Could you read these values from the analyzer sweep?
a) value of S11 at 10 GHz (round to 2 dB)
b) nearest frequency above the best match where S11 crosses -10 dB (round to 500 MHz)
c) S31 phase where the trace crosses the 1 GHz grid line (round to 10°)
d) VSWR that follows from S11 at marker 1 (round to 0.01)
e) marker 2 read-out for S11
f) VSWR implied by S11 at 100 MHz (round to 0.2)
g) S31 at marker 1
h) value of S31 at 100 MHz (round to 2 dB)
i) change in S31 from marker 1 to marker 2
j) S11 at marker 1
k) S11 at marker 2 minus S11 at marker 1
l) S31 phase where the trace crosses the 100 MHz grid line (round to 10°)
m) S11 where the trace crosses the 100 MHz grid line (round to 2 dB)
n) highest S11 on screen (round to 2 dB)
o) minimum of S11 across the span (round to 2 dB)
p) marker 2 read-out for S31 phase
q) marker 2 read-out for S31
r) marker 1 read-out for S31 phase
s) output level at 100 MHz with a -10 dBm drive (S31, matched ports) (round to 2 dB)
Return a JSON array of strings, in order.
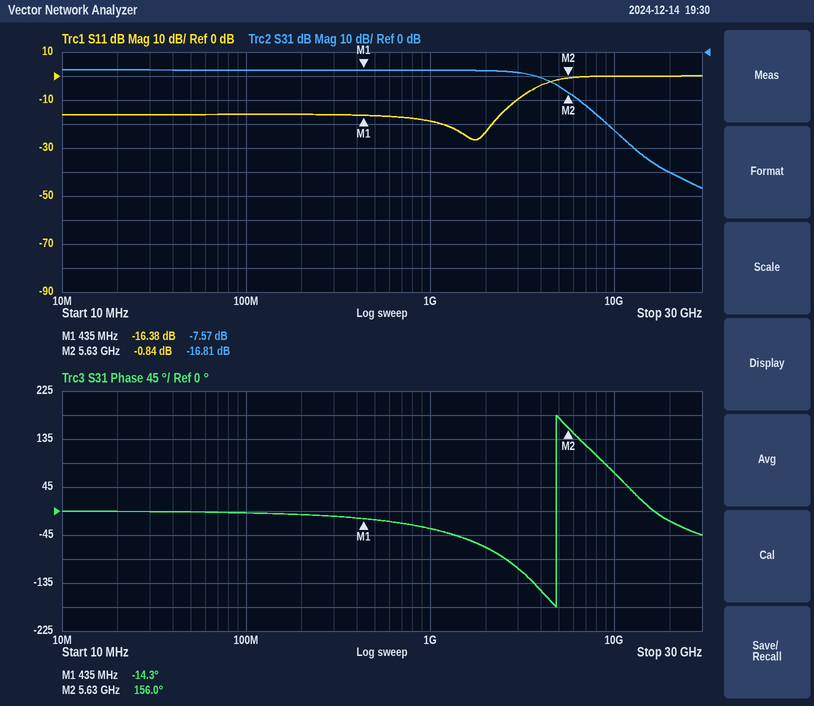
["0 dB", "3.0 GHz", "-30°", "1.36", "-0.84 dB", "1.4", "-7.57 dB", "-8 dB", "-9.24 dB", "-16.38 dB", "15.54 dB", "0°", "-16 dB", "0 dB", "-26 dB", "156.0°", "-16.81 dB", "-14.3°", "-18 dBm"]
